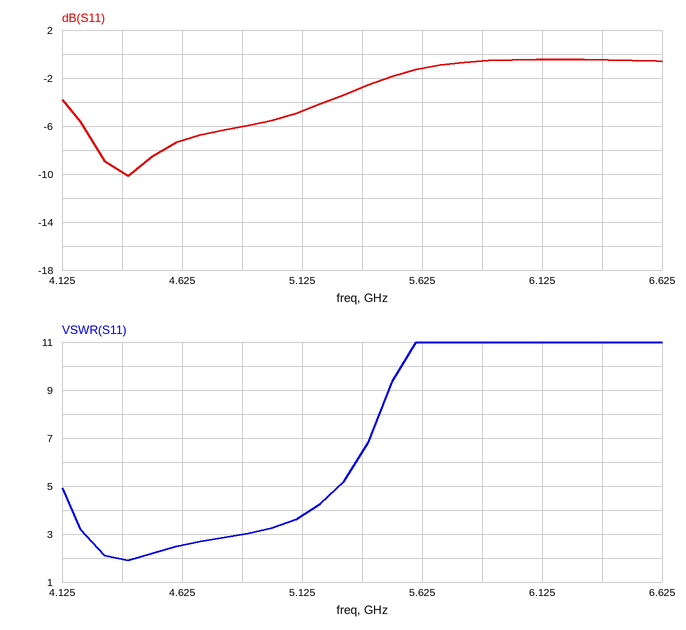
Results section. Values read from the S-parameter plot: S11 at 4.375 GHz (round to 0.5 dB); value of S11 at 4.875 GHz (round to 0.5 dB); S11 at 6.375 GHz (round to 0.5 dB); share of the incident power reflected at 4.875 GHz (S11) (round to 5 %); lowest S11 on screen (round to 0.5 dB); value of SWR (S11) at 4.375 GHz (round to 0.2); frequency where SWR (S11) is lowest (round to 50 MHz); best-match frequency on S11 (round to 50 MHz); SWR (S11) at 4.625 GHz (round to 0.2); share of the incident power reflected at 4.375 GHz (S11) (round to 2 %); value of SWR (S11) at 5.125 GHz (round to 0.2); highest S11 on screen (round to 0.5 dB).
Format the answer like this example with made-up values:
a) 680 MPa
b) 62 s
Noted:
a) -10.0 dB
b) -6.0 dB
c) -0.5 dB
d) 25 %
e) -10.0 dB
f) 2.0
g) 4.40 GHz
h) 4.40 GHz
i) 2.6
j) 10 %
k) 3.8
l) -0.5 dB
